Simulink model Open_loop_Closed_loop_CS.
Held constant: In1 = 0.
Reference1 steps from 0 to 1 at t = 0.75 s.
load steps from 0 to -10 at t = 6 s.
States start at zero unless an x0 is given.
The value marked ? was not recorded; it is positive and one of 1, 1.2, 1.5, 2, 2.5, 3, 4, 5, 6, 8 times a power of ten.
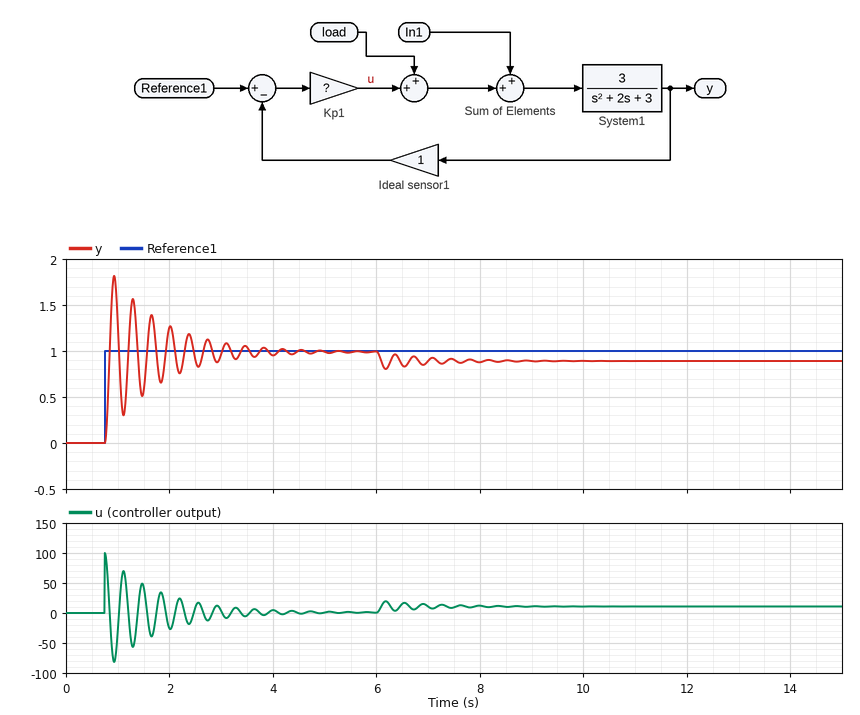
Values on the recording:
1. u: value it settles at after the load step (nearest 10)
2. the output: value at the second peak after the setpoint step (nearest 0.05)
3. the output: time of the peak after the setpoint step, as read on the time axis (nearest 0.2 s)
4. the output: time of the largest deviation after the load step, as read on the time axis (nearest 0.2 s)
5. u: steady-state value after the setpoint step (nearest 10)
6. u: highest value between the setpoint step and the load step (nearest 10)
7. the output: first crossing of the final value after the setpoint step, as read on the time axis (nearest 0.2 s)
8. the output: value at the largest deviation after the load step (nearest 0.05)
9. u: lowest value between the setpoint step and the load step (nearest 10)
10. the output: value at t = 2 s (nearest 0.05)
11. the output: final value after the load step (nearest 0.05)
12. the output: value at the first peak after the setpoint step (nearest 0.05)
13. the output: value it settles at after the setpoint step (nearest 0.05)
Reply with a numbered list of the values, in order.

1. 10
2. 1.55
3. 1.0 s
4. 6.2 s
5. 0
6. 100
7. 0.8 s
8. 0.80
9. -80
10. 1.25
11. 0.90
12. 1.80
13. 1.00
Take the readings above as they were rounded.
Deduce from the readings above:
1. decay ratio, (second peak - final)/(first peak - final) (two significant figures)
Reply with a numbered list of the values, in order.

1. 0.69
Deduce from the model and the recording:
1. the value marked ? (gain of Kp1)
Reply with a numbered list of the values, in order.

1. 100
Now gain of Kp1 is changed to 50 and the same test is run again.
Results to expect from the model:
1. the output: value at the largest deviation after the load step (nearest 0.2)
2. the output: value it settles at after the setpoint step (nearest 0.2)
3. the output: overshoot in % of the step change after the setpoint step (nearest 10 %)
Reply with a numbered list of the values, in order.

1. 0.6
2. 1.0
3. 80 %
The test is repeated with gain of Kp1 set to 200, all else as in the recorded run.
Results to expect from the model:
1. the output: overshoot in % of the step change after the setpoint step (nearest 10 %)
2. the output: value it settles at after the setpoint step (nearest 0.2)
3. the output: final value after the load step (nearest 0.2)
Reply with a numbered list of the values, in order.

1. 90 %
2. 1.0
3. 1.0
